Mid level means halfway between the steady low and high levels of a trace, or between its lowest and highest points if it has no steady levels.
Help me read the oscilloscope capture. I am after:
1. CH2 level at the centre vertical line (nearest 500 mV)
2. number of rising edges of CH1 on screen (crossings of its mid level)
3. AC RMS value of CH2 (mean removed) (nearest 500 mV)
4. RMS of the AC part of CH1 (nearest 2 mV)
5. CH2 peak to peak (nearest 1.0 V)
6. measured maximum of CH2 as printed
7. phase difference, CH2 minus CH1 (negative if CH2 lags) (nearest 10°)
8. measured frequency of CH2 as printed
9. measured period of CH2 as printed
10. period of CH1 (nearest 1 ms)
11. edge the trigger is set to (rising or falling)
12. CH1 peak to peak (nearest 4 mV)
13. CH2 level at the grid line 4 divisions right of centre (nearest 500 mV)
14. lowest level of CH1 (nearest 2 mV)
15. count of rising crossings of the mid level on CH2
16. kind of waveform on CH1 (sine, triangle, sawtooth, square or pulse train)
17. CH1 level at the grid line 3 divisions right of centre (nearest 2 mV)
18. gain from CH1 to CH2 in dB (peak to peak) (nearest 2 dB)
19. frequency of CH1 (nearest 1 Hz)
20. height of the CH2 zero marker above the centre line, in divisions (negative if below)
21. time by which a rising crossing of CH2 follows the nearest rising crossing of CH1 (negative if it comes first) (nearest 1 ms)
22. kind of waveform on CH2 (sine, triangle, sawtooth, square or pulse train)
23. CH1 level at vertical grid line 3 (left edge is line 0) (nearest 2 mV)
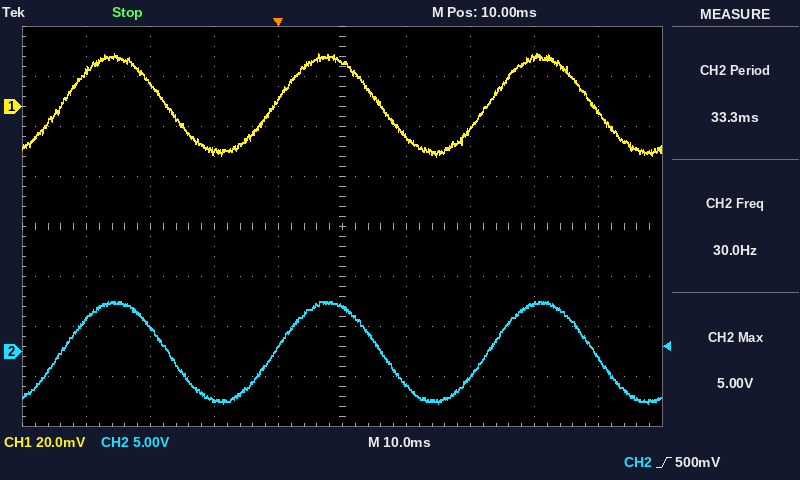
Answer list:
4.5 V
3
3.5 V
14 mV
10.0 V
5.00 V
0°
30.0 Hz
33.3 ms
33 ms
rising
40 mV
-500 mV
-20 mV
3
sine
20 mV
48 dB
30 Hz
-2.5 div
0 ms
sine
-18 mV
